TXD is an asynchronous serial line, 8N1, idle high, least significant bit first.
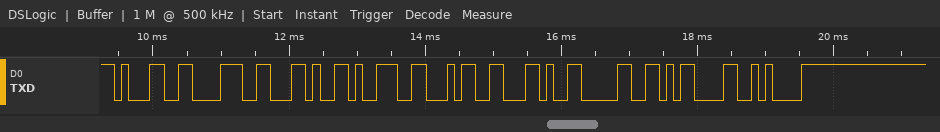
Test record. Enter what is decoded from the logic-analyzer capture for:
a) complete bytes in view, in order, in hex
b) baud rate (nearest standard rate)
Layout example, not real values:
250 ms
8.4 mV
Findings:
0x31 0x38 0x2C 0x39 0x34 0x2C 0x30 0x0D 0x0A
9600 baud
